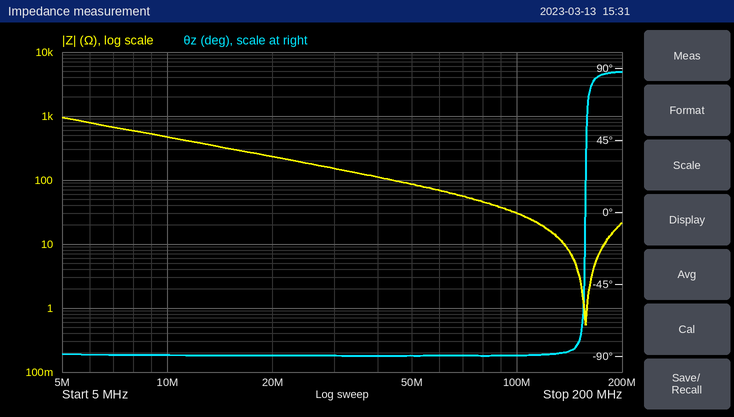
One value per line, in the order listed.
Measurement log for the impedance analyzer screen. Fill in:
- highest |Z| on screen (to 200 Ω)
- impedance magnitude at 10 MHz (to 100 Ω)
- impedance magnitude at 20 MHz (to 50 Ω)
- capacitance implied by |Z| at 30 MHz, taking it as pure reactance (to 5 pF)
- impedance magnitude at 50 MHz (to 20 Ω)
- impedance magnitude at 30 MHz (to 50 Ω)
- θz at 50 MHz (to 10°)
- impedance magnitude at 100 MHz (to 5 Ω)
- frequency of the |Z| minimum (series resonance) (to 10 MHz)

1.0 kΩ
500 Ω
250 Ω
35 pF
80 Ω
150 Ω
-90°
30 Ω
160 MHz
